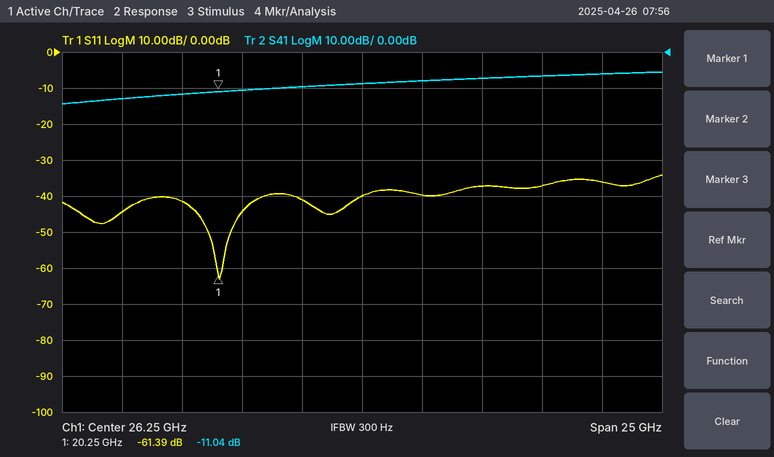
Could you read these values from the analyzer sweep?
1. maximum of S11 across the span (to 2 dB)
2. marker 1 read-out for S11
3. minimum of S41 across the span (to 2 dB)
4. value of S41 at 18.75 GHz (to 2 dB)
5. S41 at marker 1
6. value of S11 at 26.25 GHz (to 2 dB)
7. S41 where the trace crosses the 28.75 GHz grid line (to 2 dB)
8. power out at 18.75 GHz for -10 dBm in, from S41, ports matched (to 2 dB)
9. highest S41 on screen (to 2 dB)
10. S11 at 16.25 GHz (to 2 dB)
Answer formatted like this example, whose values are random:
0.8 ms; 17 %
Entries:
-34 dB; -61.39 dB; -14 dB; -12 dB; -11.04 dB; -40 dB; -8 dB; -22 dBm; -6 dB; -44 dB
